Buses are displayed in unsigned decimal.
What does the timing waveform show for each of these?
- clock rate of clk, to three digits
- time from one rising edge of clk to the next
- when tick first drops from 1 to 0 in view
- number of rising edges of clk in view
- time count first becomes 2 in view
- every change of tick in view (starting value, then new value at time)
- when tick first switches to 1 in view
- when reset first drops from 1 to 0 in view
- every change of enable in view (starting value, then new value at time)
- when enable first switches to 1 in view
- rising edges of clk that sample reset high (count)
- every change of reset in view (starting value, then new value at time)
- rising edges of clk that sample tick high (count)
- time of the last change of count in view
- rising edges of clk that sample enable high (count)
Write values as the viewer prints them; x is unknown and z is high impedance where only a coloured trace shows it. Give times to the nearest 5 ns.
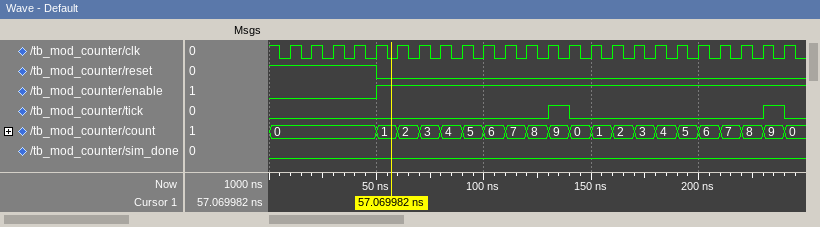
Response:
100 MHz
10 ns
140 ns
24
60 ns
0, 1 at 130 ns, 0 at 140 ns, 1 at 230 ns, 0 at 240 ns
130 ns
50 ns
0, 1 at 50 ns
50 ns
5
1, 0 at 50 ns
2
240 ns
19
